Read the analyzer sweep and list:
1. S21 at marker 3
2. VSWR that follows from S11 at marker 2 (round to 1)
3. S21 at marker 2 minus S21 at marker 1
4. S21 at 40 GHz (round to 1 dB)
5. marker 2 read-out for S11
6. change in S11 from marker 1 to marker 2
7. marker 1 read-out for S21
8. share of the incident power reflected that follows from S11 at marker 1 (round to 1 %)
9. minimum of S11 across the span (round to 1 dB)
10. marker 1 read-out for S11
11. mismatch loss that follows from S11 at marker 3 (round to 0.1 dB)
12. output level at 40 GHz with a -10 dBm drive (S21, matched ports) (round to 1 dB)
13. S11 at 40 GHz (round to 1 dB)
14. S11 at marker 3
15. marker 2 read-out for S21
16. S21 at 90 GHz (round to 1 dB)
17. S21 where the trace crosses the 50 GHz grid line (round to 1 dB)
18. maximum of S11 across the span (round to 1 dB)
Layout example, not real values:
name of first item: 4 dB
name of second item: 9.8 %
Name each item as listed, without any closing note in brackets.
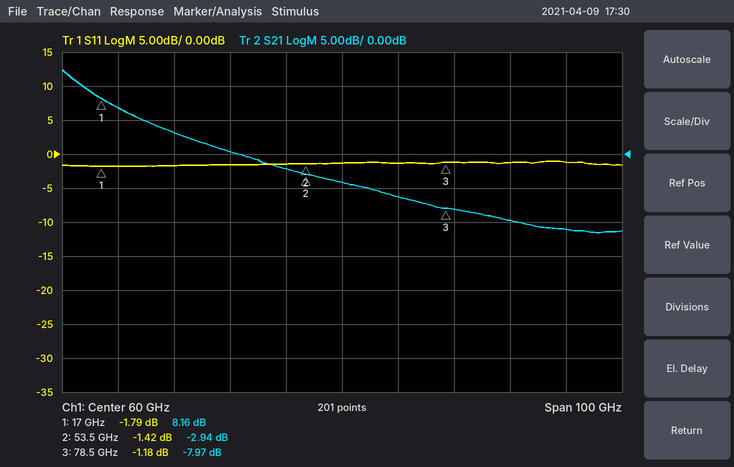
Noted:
S21 at marker 3: -7.97 dB
VSWR that follows from S11 at marker 2: 12
S21 at marker 2 minus S21 at marker 1: -11.10 dB
S21 at 40 GHz: 0 dB
marker 2 read-out for S11: -1.42 dB
change in S11 from marker 1 to marker 2: 0.37 dB
marker 1 read-out for S21: 8.16 dB
share of the incident power reflected that follows from S11 at marker 1: 66 %
minimum of S11 across the span: -2 dB
marker 1 read-out for S11: -1.79 dB
mismatch loss that follows from S11 at marker 3: 6.2 dB
output level at 40 GHz with a -10 dBm drive (S21, matched ports): -10 dBm
S11 at 40 GHz: -2 dB
S11 at marker 3: -1.18 dB
marker 2 read-out for S21: -2.94 dB
S21 at 90 GHz: -10 dB
S21 where the trace crosses the 50 GHz grid line: -2 dB
maximum of S11 across the span: -1 dB
